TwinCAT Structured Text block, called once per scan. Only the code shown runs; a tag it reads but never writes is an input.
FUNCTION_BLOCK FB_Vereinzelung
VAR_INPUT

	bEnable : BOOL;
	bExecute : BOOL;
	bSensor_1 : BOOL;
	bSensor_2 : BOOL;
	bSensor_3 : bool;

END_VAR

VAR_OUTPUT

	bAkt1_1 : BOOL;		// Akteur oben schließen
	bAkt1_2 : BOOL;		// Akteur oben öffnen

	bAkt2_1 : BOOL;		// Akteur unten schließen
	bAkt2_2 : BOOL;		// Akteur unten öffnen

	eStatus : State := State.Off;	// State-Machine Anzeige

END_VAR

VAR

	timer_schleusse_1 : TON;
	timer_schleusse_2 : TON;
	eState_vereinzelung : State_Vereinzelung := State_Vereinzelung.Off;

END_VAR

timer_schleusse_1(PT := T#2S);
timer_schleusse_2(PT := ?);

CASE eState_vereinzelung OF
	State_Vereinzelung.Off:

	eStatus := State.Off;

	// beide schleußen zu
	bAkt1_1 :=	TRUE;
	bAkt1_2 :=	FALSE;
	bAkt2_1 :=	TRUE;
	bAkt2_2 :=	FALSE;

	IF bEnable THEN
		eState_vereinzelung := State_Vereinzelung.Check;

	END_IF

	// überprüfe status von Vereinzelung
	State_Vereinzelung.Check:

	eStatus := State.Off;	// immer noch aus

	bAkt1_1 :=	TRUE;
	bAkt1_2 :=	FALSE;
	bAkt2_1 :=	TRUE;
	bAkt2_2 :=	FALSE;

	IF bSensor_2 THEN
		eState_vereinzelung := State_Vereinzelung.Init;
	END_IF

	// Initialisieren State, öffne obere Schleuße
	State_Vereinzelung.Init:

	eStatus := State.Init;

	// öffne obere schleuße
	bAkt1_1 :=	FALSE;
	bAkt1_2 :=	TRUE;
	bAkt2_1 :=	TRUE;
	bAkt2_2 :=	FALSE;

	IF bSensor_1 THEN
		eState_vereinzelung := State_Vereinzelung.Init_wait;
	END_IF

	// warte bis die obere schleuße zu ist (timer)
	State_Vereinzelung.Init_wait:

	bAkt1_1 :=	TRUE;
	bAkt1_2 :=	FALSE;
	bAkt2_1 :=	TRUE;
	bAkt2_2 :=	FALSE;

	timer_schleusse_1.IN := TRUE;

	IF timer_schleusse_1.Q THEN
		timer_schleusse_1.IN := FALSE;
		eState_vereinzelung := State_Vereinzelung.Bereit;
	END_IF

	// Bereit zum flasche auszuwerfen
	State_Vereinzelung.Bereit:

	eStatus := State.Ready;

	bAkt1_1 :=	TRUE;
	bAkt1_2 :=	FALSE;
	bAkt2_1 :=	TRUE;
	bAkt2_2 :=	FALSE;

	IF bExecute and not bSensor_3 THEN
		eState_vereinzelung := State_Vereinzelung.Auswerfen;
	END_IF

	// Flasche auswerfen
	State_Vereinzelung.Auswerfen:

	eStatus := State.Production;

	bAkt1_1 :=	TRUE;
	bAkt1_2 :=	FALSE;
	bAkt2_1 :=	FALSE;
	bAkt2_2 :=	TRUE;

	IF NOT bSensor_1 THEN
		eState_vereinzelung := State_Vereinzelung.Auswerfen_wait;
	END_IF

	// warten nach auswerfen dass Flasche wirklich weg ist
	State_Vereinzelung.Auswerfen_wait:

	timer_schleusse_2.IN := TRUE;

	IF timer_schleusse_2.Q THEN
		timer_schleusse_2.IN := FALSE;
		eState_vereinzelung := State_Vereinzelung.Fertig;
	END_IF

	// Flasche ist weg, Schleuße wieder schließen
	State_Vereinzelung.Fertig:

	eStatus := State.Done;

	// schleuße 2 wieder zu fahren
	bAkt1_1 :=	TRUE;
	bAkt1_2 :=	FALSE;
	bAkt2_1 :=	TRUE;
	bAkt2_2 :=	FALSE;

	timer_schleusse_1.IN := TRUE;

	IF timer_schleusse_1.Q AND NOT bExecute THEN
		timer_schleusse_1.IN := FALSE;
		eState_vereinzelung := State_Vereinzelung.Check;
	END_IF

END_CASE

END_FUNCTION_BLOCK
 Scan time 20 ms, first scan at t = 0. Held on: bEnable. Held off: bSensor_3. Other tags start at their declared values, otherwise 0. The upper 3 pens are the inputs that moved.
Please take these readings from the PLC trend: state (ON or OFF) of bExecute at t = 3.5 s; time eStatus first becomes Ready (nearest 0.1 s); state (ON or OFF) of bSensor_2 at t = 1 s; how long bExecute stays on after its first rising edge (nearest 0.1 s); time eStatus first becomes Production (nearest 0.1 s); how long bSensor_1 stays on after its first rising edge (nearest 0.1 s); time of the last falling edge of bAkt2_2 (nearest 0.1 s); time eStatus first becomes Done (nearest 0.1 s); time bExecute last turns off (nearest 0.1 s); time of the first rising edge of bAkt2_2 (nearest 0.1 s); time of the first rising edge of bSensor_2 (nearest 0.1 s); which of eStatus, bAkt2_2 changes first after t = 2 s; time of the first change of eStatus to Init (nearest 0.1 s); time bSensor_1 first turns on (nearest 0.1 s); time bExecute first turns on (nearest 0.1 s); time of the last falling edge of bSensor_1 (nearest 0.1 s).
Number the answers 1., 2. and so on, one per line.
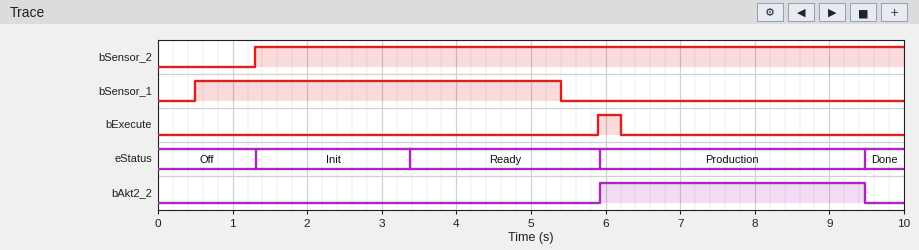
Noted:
1. OFF
2. 3.4 s
3. OFF
4. 0.3 s
5. 5.9 s
6. 4.9 s
7. 9.5 s
8. 9.5 s
9. 6.2 s
10. 5.9 s
11. 1.3 s
12. eStatus
13. 1.3 s
14. 0.5 s
15. 5.9 s
16. 5.4 s
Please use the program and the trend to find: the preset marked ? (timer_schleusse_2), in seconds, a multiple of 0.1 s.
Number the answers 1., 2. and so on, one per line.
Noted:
1. 3.5 s
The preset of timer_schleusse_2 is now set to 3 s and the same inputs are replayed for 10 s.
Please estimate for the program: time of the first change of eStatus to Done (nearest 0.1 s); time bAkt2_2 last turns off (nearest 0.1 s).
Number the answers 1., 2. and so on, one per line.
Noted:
1. 9.0 s
2. 9.0 s
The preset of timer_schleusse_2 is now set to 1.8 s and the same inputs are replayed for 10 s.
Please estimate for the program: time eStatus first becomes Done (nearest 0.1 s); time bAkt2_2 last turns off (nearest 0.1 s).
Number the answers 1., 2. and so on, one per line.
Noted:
1. 7.8 s
2. 7.8 s
